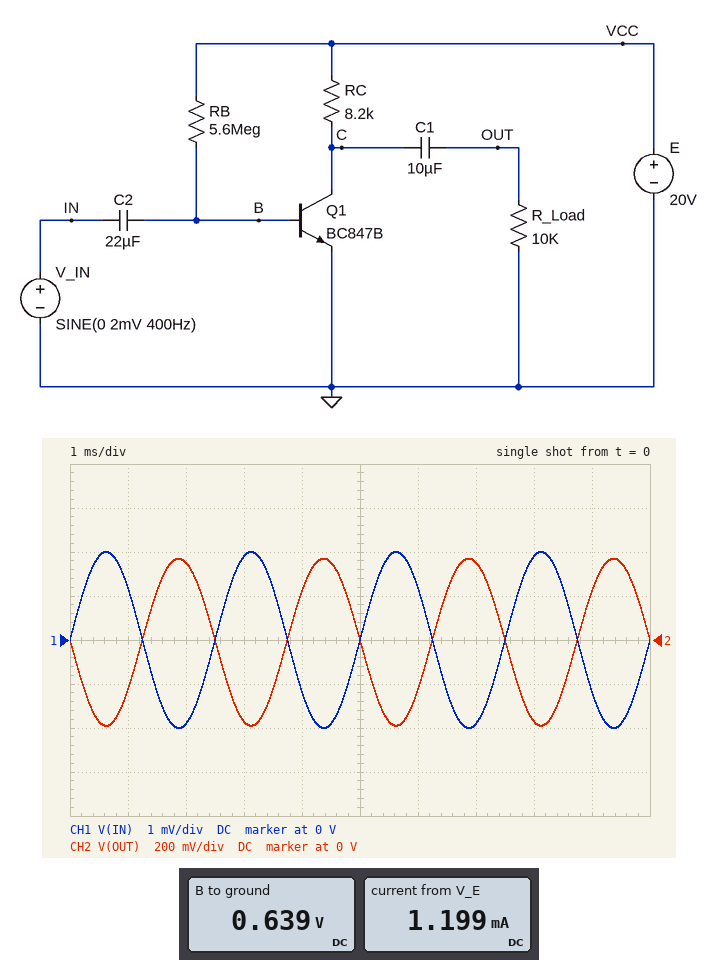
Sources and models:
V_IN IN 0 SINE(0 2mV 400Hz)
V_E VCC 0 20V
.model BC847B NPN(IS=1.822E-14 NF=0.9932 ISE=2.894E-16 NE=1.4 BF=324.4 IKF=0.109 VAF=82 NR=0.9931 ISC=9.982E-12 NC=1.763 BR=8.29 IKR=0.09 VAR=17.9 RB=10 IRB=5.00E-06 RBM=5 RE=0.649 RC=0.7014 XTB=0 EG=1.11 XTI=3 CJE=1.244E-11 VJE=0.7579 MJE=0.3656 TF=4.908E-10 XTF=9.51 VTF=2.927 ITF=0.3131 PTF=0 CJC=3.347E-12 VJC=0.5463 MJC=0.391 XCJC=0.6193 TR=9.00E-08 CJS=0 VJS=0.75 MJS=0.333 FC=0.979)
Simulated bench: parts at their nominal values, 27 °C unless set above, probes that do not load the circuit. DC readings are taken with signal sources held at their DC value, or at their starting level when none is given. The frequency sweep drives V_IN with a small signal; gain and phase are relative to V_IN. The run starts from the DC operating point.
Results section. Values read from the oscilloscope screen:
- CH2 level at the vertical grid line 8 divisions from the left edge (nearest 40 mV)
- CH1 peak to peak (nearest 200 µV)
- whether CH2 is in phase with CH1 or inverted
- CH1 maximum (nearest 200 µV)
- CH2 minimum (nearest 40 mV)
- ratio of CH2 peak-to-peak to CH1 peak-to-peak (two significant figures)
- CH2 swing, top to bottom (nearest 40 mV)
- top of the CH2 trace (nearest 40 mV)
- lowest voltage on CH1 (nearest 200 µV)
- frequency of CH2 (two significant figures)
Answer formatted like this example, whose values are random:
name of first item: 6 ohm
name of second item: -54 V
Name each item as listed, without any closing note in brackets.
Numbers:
CH2 level at the vertical grid line 8 divisions from the left edge: -360 mV
CH1 peak to peak: 4.0 mV
whether CH2 is in phase with CH1 or inverted: inverted
CH1 maximum: 2.0 mV
CH2 minimum: -400 mV
ratio of CH2 peak-to-peak to CH1 peak-to-peak: 190
CH2 swing, top to bottom: 760 mV
top of the CH2 trace: 360 mV
lowest voltage on CH1: -2.0 mV
frequency of CH2: 400 Hz
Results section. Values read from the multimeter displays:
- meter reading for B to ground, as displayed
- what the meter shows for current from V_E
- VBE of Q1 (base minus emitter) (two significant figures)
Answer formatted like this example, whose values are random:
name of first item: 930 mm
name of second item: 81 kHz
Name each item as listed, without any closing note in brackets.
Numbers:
meter reading for B to ground, as displayed: 0.639 V
what the meter shows for current from V_E: 1.199 mA
VBE of Q1 (base minus emitter): 640 mV
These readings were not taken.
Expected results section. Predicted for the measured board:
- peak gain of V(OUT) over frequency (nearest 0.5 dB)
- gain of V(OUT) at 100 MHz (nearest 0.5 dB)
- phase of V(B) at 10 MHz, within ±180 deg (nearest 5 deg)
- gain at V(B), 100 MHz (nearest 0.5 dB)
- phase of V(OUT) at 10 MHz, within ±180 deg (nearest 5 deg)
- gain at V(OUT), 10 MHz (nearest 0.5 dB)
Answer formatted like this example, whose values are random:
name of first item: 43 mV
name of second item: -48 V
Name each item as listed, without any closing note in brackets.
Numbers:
peak gain of V(OUT) over frequency: 45.5 dB
gain of V(OUT) at 100 MHz: 34.0 dB
phase of V(B) at 10 MHz, within ±180 deg: 0 deg
gain at V(B), 100 MHz: 0 dB
phase of V(OUT) at 10 MHz, within ±180 deg: 160 deg
gain at V(OUT), 10 MHz: 45.0 dB
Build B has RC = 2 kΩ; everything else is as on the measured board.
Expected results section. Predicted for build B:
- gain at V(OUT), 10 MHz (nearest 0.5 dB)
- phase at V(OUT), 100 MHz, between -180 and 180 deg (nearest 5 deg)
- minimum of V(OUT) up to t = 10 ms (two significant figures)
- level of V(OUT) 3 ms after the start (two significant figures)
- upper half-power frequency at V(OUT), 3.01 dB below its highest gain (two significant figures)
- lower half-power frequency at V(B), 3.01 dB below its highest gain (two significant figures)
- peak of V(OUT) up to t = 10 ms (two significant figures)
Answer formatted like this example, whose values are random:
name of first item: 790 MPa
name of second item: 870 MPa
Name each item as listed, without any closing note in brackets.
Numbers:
gain at V(OUT), 10 MHz: 38.0 dB
phase at V(OUT), 100 MHz, between -180 and 180 deg: 120 deg
minimum of V(OUT) up to t = 10 ms: -160 mV
level of V(OUT) 3 ms after the start: -150 mV
upper half-power frequency at V(OUT), 3.01 dB below its highest gain: 85 MHz
lower half-power frequency at V(B), 3.01 dB below its highest gain: 940 mHz
peak of V(OUT) up to t = 10 ms: 150 mV
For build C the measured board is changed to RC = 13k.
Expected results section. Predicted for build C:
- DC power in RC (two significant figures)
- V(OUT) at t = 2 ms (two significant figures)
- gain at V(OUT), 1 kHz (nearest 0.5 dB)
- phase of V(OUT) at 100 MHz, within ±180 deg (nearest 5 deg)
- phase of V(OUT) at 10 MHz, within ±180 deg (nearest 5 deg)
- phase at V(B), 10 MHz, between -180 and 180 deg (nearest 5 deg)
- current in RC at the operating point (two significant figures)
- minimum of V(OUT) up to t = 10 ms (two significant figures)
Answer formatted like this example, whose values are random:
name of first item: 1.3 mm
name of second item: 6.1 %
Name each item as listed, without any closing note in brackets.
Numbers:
DC power in RC: 17 mW
V(OUT) at t = 2 ms: 410 mV
gain at V(OUT), 1 kHz: 47.0 dB
phase of V(OUT) at 100 MHz, within ±180 deg: 90 deg
phase of V(OUT) at 10 MHz, within ±180 deg: 150 deg
phase at V(B), 10 MHz, between -180 and 180 deg: 0 deg
current in RC at the operating point: 1.1 mA
minimum of V(OUT) up to t = 10 ms: -460 mV
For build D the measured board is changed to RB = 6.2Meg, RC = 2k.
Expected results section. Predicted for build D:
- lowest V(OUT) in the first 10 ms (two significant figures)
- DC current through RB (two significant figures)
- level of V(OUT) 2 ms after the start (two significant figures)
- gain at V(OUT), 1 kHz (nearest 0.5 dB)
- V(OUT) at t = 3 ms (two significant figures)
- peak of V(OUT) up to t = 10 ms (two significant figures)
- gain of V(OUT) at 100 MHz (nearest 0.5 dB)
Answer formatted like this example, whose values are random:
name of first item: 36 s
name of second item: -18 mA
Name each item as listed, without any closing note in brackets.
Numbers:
lowest V(OUT) in the first 10 ms: -150 mV
DC current through RB: 3.1 µA
level of V(OUT) 2 ms after the start: 130 mV
gain at V(OUT), 1 kHz: 37.0 dB
V(OUT) at t = 3 ms: -140 mV
peak of V(OUT) up to t = 10 ms: 140 mV
gain of V(OUT) at 100 MHz: 33.5 dB
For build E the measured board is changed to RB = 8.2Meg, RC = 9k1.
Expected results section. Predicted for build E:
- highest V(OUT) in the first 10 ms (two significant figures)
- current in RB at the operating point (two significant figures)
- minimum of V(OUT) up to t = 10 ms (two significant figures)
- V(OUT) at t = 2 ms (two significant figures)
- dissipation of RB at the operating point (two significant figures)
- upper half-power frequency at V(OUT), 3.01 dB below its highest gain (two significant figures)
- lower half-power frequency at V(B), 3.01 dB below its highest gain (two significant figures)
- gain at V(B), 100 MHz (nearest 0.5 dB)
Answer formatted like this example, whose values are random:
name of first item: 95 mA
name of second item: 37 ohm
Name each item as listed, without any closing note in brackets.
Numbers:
highest V(OUT) in the first 10 ms: 280 mV
current in RB at the operating point: 2.4 µA
minimum of V(OUT) up to t = 10 ms: -300 mV
V(OUT) at t = 2 ms: 270 mV
dissipation of RB at the operating point: 46 µW
upper half-power frequency at V(OUT), 3.01 dB below its highest gain: 30 MHz
lower half-power frequency at V(B), 3.01 dB below its highest gain: 650 mHz
gain at V(B), 100 MHz: 0 dB
